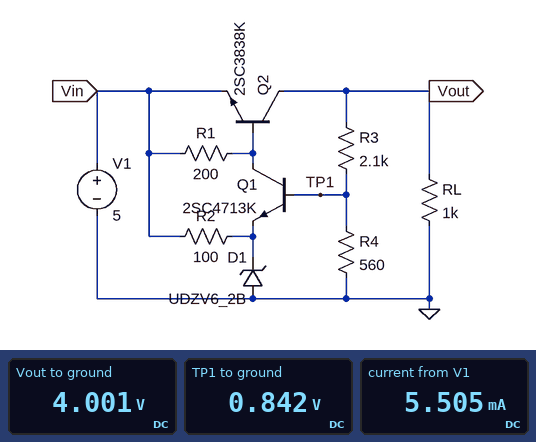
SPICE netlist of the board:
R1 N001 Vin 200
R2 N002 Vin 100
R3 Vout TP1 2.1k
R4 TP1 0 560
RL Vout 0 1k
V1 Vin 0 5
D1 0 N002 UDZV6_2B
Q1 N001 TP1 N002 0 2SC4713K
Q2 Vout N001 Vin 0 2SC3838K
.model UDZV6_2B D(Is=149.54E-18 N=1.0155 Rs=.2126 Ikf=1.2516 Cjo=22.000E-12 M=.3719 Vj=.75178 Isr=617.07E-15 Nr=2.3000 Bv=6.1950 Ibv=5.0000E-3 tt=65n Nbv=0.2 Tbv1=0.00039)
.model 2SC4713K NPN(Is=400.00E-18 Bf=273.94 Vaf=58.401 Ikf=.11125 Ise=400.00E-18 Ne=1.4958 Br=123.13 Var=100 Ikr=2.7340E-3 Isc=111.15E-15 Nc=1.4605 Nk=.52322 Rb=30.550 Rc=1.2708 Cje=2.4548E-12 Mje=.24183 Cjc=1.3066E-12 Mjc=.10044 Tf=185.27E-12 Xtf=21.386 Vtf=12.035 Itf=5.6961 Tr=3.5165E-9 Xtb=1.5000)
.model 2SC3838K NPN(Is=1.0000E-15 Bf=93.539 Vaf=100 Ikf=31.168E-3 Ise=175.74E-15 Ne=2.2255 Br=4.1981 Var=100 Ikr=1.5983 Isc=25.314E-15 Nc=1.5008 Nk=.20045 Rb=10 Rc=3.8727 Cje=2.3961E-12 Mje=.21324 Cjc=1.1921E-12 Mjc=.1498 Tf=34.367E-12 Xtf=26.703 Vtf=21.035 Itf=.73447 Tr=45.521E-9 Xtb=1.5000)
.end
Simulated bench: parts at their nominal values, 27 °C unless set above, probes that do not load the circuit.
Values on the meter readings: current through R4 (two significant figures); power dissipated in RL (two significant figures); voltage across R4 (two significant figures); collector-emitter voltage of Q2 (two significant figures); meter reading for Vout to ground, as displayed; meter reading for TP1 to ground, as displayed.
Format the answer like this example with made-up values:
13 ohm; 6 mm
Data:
1.5 mA; 16 mW; 840 mV; -1.0 V; 4.001 V; 0.842 V
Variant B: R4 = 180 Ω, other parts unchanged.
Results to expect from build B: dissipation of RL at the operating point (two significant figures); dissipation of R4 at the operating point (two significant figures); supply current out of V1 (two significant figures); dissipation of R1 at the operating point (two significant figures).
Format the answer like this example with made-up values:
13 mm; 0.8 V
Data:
16 mW; 550 µW; 5.7 mA; 250 µW
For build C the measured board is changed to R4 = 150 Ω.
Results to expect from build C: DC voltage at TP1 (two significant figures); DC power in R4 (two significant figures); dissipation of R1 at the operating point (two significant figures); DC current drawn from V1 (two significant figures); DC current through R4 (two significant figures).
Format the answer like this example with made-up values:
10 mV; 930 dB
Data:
270 mV; 470 µW; 250 µW; 5.8 mA; 1.8 mA
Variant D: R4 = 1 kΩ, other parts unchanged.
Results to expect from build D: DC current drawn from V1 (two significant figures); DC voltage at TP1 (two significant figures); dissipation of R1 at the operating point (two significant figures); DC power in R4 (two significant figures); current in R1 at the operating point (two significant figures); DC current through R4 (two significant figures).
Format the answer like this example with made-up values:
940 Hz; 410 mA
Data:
5.3 mA; 1.3 V; 210 µW; 1.7 mW; 1.0 mA; 1.3 mA
